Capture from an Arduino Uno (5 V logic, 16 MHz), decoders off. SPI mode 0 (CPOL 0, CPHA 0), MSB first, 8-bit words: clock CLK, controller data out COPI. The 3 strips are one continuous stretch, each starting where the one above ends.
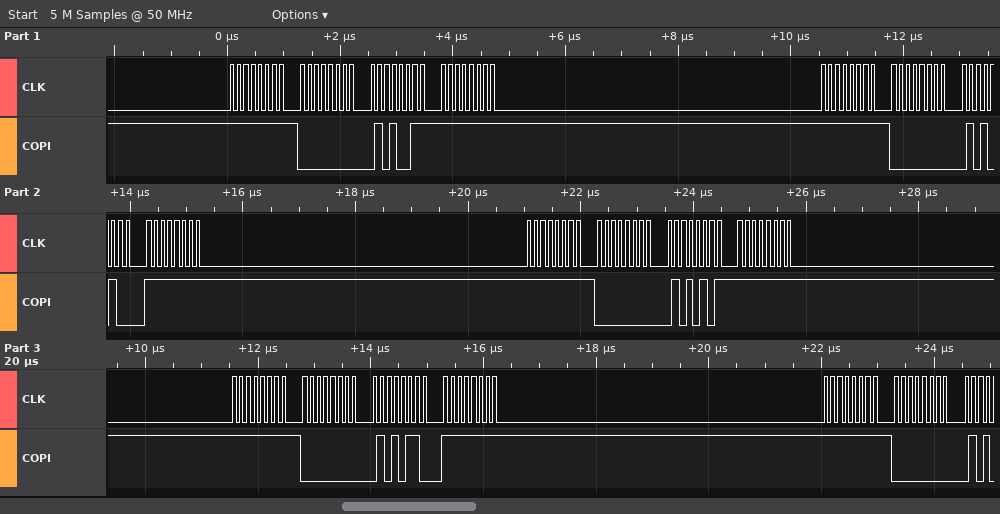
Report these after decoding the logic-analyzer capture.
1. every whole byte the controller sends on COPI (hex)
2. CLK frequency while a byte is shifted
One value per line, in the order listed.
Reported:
FF 00 53 FF FF 00 54 FF FF 00 55 FF FF 00 56 FF FF 00
8 MHz
